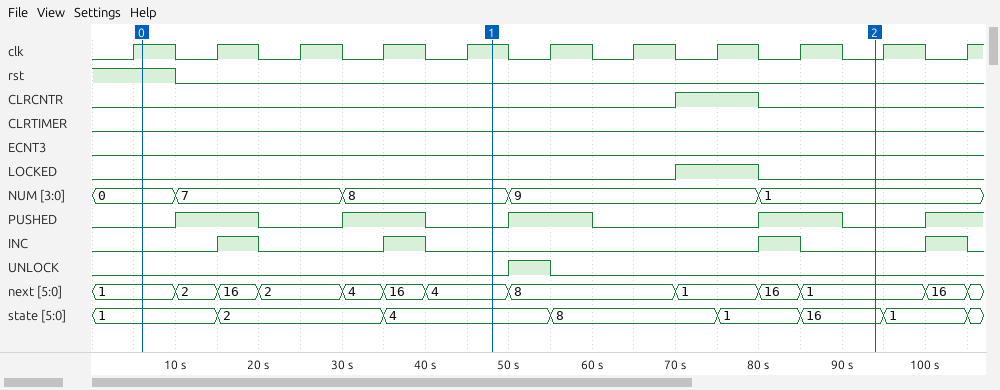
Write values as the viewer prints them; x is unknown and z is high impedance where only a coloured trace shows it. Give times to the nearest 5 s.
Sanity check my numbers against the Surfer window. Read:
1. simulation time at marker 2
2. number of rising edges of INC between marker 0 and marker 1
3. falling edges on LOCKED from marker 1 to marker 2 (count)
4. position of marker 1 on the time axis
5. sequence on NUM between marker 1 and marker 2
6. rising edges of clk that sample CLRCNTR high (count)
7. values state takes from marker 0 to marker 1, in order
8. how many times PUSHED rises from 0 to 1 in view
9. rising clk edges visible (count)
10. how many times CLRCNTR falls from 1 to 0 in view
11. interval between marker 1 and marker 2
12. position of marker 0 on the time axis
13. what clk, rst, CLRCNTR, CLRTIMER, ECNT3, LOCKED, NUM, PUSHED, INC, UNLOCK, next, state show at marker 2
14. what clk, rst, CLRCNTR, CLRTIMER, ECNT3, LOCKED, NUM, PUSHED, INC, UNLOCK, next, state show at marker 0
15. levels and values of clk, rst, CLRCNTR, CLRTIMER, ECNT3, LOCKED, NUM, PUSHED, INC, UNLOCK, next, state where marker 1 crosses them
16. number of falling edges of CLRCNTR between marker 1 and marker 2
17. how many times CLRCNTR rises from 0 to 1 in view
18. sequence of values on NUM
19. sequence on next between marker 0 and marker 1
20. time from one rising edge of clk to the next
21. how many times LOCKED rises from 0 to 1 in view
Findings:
95 s
2
1
50 s
8, 9, 1
1
1, 2, 4
5
11
1
45 s
5 s
clk=0, rst=0, CLRCNTR=0, CLRTIMER=0, ECNT3=0, LOCKED=0, NUM=1, PUSHED=0, INC=0, UNLOCK=0, next=1, state=16
clk=1, rst=1, CLRCNTR=0, CLRTIMER=0, ECNT3=0, LOCKED=0, NUM=0, PUSHED=0, INC=0, UNLOCK=0, next=1, state=1
clk=1, rst=0, CLRCNTR=0, CLRTIMER=0, ECNT3=0, LOCKED=0, NUM=8, PUSHED=0, INC=0, UNLOCK=0, next=4, state=4
1
1
0, 7, 8, 9, 1
1, 2, 16, 2, 4, 16, 4
10 s
1
